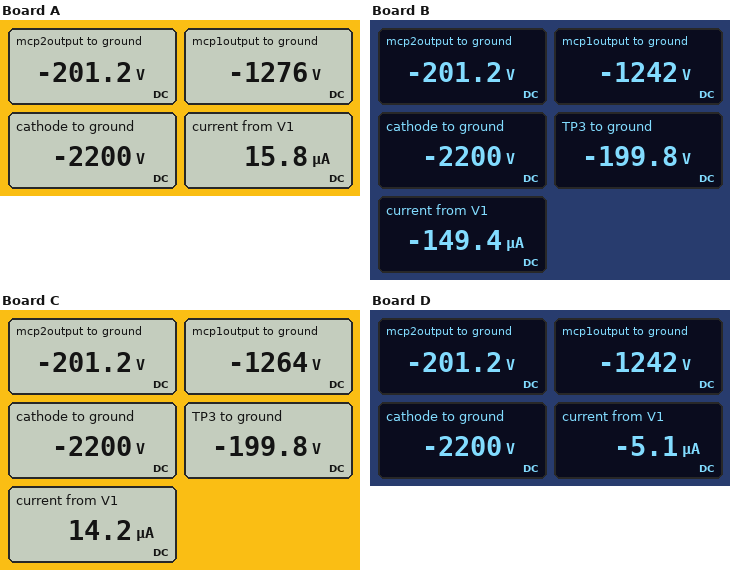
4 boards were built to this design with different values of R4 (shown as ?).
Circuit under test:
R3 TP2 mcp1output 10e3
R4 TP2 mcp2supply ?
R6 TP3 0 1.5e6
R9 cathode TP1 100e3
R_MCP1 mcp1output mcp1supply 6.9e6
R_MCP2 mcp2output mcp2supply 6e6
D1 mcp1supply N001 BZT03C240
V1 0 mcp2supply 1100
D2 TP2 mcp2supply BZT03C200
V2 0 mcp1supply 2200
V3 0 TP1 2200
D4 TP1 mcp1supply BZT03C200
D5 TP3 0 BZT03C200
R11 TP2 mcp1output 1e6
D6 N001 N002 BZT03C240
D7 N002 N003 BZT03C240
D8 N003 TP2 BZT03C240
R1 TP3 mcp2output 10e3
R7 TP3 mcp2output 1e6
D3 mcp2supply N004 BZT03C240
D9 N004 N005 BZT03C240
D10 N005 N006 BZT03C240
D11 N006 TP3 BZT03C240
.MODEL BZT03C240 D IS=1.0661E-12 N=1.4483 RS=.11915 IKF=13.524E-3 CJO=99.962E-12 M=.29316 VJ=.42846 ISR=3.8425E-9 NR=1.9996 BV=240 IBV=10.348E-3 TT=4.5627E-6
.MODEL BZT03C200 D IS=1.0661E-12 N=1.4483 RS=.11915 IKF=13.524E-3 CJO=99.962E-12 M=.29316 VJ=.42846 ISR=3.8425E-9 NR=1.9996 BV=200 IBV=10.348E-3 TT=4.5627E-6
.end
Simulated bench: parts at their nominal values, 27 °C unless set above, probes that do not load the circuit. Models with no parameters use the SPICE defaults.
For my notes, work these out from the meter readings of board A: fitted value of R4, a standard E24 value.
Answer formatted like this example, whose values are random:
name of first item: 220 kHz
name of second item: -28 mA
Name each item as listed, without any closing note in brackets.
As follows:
fitted value of R4, a standard E24 value: 1.3 MΩ
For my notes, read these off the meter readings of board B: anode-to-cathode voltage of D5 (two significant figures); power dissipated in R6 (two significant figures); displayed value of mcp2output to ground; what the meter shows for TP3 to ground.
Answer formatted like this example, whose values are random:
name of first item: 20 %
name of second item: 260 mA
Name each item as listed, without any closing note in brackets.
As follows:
anode-to-cathode voltage of D5: -200 V
power dissipated in R6: 27 mW
displayed value of mcp2output to ground: -201.2 V
what the meter shows for TP3 to ground: -199.8 V
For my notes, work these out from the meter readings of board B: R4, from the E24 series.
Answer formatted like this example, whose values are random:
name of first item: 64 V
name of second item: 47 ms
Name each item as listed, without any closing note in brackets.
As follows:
R4, from the E24 series: 470 kΩ
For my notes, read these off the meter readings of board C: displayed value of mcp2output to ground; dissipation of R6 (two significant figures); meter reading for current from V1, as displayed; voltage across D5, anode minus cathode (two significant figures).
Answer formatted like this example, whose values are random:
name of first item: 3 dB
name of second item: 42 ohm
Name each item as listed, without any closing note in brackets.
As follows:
displayed value of mcp2output to ground: -201.2 V
dissipation of R6: 27 mW
meter reading for current from V1, as displayed: 14.2 µA
voltage across D5, anode minus cathode: -200 V
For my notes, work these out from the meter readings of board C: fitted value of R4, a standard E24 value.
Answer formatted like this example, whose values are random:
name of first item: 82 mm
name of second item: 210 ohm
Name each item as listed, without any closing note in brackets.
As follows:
fitted value of R4, a standard E24 value: 1.2 MΩ
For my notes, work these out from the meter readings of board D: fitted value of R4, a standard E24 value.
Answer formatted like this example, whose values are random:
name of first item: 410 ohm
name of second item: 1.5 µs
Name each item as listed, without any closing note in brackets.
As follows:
fitted value of R4, a standard E24 value: 910 kΩ
